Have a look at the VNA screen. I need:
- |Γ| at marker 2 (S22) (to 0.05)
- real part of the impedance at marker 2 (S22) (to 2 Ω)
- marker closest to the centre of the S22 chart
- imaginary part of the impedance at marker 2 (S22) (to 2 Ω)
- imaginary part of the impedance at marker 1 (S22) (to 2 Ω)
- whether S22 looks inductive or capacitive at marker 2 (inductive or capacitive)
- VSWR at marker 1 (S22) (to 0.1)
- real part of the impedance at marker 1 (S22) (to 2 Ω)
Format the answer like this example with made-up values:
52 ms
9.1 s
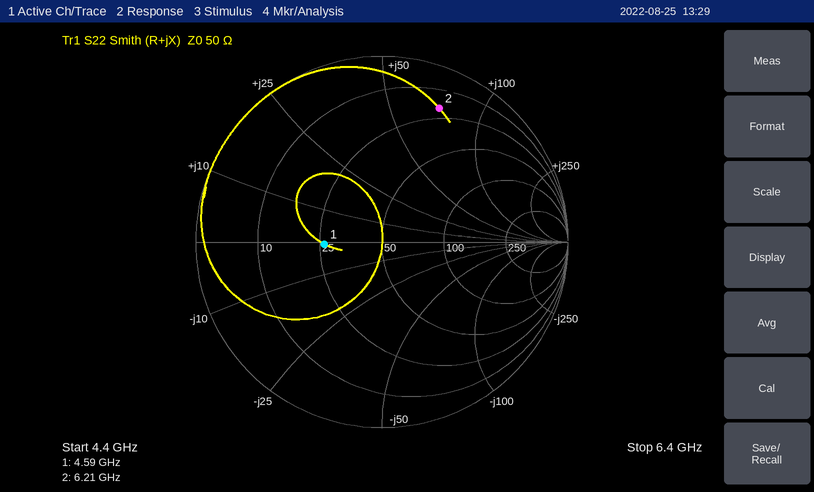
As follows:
0.80
20 Ω
marker 1
+72 Ω
0 Ω
inductive
1.9
26 Ω
